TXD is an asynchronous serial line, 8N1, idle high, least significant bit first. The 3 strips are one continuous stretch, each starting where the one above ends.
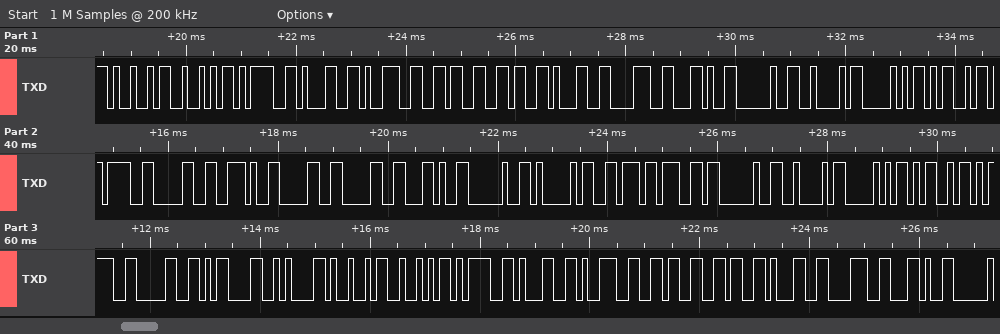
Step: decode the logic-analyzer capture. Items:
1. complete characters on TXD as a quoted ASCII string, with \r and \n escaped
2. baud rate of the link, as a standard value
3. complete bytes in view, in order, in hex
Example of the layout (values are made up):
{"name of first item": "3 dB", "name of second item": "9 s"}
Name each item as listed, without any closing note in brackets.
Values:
{"complete characters on TXD as a quoted ASCII string, with \\r and \\n escaped": "\"IR=196618, BPM=0.00, Avg BPM=0\\r\\nIR=196618,\"", "baud rate of the link, as a standard value": "9600 baud", "complete bytes in view, in order, in hex": "49 52 3D 31 39 36 36 31 38 2C 20 42 50 4D 3D 30 2E 30 30 2C 20 41 76 67 20 42 50 4D 3D 30 0D 0A 49 52 3D 31 39 36 36 31 38 2C"}
